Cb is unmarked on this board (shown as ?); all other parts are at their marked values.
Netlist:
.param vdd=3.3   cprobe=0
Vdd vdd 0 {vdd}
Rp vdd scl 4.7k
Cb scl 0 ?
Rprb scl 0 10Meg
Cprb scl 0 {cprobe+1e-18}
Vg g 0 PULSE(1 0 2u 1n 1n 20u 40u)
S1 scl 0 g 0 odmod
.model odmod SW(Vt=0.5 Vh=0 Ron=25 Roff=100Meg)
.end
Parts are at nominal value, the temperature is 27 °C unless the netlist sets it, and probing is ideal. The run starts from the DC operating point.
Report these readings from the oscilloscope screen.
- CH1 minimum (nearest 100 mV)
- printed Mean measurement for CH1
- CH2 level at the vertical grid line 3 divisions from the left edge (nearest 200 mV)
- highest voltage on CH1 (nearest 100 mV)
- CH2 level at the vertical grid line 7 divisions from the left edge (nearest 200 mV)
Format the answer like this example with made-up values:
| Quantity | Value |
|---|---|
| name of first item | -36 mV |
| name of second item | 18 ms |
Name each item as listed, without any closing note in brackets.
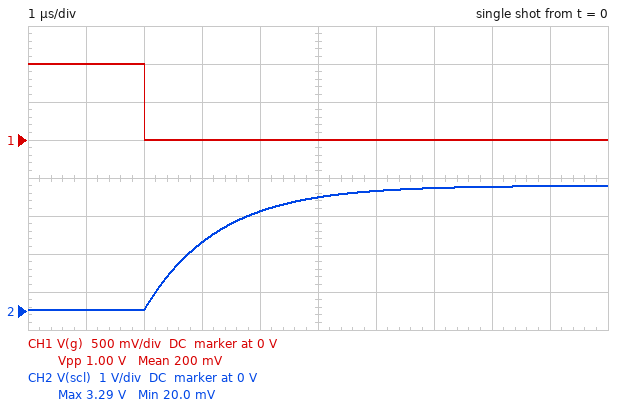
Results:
| Quantity | Value |
|---|---|
| CH1 minimum | 0 V |
| printed Mean measurement for CH1 | 200 mV |
| CH2 level at the vertical grid line 3 divisions from the left edge | 1.8 V |
| highest voltage on CH1 | 1.0 V |
| CH2 level at the vertical grid line 7 divisions from the left edge | 3.2 V |
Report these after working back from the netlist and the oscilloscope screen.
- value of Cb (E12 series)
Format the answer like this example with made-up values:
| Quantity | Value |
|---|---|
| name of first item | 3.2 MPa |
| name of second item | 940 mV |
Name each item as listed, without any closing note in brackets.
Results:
| Quantity | Value |
|---|---|
| value of Cb | 270 pF |
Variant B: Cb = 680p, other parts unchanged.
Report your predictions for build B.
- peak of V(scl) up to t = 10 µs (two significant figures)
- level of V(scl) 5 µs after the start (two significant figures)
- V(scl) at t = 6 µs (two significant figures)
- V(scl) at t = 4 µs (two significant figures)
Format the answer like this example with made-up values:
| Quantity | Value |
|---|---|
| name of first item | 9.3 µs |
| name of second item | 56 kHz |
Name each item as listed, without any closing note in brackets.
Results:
| Quantity | Value |
|---|---|
| peak of V(scl) up to t = 10 µs | 3.0 V |
| level of V(scl) 5 µs after the start | 2.0 V |
| V(scl) at t = 6 µs | 2.4 V |
| V(scl) at t = 4 µs | 1.5 V |
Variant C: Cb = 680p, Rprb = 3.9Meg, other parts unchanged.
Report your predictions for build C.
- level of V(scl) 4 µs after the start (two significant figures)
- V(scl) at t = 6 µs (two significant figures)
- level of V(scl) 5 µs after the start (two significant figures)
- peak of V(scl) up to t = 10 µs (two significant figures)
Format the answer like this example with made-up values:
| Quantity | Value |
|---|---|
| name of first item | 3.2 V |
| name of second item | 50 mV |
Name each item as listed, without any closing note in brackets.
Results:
| Quantity | Value |
|---|---|
| level of V(scl) 4 µs after the start | 1.5 V |
| V(scl) at t = 6 µs | 2.4 V |
| level of V(scl) 5 µs after the start | 2.0 V |
| peak of V(scl) up to t = 10 µs | 3.0 V |
